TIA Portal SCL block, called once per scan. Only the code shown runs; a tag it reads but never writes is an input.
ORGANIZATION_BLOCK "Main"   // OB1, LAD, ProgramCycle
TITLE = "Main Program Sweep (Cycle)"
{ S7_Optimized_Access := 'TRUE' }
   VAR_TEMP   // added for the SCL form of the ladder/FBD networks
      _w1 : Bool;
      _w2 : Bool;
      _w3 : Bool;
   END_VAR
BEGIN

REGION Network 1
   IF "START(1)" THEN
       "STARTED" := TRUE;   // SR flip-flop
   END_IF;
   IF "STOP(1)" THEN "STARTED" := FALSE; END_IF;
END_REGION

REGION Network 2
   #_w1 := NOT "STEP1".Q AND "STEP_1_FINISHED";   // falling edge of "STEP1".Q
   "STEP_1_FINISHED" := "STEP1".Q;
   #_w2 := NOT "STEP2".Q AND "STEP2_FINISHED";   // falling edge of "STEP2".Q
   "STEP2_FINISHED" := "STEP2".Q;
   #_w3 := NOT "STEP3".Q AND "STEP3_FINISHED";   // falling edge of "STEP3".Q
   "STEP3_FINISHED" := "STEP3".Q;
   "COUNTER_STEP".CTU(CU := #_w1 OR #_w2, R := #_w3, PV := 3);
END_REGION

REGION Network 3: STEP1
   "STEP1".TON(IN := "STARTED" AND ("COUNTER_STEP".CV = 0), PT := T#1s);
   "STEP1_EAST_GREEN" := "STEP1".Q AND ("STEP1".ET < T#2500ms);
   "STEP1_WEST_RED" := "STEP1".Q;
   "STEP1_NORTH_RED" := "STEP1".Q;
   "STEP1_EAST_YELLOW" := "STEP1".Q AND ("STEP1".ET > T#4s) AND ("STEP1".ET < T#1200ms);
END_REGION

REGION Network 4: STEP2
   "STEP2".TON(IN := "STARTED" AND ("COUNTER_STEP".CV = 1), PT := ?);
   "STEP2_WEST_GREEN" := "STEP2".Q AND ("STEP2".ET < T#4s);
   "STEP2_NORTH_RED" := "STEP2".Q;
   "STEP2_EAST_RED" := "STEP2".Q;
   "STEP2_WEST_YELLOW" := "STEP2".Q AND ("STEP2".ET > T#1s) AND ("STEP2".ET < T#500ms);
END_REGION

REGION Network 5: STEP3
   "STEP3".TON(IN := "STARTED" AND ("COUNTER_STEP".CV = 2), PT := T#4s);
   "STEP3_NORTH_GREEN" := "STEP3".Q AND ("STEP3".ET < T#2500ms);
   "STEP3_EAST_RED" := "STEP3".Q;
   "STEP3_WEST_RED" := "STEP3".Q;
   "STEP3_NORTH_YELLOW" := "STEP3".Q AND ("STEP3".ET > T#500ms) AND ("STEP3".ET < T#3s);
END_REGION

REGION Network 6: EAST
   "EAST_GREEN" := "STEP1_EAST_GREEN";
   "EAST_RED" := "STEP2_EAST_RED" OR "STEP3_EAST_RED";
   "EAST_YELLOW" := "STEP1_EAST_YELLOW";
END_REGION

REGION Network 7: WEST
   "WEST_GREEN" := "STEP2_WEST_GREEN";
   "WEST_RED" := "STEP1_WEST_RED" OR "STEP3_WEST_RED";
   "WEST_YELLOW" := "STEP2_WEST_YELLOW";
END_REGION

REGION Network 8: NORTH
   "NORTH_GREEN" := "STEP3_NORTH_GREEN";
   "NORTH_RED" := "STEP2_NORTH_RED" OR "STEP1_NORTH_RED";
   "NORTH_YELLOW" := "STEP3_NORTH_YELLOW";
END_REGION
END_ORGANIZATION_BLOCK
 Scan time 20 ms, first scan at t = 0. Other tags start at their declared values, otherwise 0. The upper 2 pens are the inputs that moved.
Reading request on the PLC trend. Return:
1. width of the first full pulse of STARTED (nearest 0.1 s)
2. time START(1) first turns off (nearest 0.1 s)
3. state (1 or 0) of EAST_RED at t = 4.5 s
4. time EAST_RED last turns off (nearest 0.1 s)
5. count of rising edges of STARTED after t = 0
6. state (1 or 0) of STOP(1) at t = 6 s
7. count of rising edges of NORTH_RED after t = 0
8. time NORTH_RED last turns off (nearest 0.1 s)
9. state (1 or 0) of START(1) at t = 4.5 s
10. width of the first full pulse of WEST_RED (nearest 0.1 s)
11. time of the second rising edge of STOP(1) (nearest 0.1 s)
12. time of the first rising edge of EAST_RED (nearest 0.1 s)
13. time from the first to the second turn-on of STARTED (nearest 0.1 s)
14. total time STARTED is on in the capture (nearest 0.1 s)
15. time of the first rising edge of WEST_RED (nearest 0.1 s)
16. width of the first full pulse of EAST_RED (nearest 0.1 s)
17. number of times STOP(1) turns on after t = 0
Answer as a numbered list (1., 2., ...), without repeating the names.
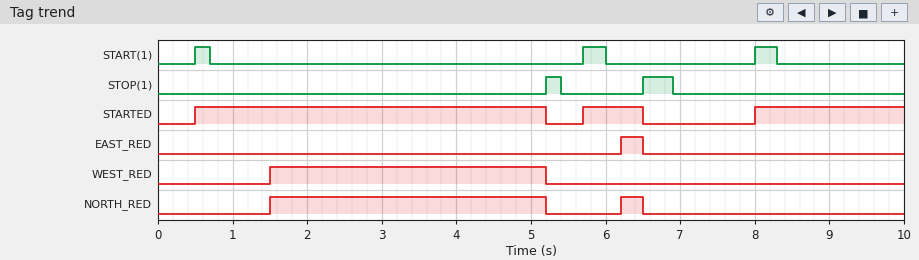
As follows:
1. 4.7 s
2. 0.7 s
3. 0
4. 6.5 s
5. 3
6. 0
7. 2
8. 6.5 s
9. 0
10. 3.7 s
11. 6.5 s
12. 6.2 s
13. 5.2 s
14. 7.5 s
15. 1.5 s
16. 0.3 s
17. 2
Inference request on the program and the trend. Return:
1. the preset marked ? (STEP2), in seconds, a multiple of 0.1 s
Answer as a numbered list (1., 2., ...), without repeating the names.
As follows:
1. 0.5 s
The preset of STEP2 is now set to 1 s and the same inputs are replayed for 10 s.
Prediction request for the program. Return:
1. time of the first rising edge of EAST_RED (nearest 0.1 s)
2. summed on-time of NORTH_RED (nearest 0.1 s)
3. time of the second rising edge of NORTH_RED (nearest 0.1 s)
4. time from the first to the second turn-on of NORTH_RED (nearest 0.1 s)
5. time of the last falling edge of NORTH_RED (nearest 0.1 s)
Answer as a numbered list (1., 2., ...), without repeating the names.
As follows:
1. 9.0 s
2. 4.7 s
3. 9.0 s
4. 7.5 s
5. 5.2 s
